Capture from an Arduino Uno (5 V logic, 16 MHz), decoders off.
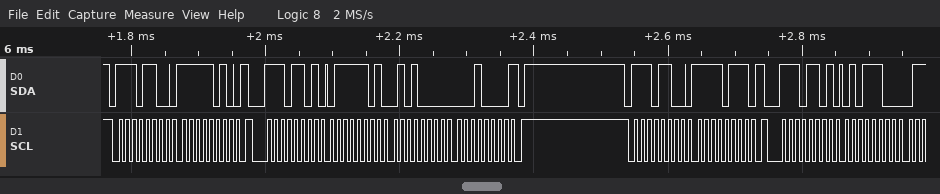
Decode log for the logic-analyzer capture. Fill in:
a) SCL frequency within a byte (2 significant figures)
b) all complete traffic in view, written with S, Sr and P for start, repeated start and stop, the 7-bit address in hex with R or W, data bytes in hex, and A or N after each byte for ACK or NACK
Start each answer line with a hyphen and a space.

- 100 kHz
- S 76W A FA A Sr 76R A 7D A 50 A 10 N P S 76W A F7 A Sr 76R A 5C A
